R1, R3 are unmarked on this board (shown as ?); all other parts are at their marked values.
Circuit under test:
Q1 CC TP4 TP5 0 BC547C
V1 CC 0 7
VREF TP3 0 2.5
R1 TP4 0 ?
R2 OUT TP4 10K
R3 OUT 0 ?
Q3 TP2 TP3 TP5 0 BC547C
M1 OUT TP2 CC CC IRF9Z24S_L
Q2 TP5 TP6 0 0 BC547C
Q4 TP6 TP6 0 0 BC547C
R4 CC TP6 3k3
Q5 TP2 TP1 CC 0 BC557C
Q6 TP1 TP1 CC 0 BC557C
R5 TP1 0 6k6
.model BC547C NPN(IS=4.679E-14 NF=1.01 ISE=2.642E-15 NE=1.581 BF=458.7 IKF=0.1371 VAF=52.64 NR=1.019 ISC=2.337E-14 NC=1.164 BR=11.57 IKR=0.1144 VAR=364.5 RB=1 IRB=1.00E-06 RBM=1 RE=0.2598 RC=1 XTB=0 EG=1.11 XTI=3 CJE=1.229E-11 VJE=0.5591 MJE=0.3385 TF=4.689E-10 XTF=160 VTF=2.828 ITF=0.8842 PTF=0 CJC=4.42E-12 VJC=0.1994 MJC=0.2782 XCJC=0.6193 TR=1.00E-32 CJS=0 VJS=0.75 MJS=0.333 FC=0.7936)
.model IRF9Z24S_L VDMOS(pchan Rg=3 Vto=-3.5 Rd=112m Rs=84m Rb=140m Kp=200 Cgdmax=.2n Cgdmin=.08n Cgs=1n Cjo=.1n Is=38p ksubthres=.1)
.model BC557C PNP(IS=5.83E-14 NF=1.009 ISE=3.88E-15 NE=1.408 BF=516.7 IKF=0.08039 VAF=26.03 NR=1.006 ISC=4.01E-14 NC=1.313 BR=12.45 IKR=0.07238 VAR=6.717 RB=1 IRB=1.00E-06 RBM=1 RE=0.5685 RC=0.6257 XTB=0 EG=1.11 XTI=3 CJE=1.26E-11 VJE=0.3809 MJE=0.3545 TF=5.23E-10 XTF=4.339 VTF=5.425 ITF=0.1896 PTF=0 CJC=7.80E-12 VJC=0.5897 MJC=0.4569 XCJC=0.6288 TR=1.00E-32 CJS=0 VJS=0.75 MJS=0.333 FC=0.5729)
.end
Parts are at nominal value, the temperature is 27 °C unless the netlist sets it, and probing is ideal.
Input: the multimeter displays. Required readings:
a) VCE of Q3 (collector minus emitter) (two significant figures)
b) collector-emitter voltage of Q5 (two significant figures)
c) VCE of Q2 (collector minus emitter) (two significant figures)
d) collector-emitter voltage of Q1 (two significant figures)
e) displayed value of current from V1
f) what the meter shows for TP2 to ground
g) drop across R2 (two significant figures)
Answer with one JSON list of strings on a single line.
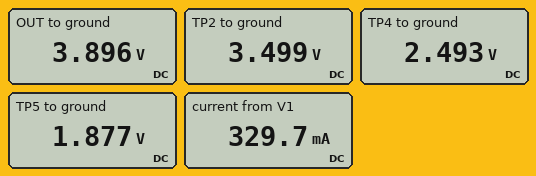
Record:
["1.6 V", "-3.5 V", "1.9 V", "5.1 V", "329.7 mA", "3.499 V", "1.4 V"]
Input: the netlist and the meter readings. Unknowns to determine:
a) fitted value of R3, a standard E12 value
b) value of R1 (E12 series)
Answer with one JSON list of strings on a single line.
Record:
["12 Ω", "18 kΩ"]
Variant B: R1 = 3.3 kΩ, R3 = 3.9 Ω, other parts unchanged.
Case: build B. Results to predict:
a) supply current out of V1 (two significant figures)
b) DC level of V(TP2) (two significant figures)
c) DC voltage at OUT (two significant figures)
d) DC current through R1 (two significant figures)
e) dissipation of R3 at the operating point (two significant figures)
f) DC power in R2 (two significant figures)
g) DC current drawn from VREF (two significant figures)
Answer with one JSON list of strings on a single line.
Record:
["1.7 A", "1.8 V", "6.7 V", "500 µA", "11 W", "2.5 mW", "820 µA"]
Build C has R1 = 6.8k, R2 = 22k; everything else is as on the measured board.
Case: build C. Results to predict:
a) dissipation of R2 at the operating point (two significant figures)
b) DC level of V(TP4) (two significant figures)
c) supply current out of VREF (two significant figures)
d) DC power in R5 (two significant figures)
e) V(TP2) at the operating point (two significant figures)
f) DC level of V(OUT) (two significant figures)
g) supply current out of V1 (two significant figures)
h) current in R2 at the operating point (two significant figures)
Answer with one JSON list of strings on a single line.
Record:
["1.3 mW", "1.6 V", "820 µA", "6.2 mW", "1.8 V", "6.9 V", "580 mA", "240 µA"]
